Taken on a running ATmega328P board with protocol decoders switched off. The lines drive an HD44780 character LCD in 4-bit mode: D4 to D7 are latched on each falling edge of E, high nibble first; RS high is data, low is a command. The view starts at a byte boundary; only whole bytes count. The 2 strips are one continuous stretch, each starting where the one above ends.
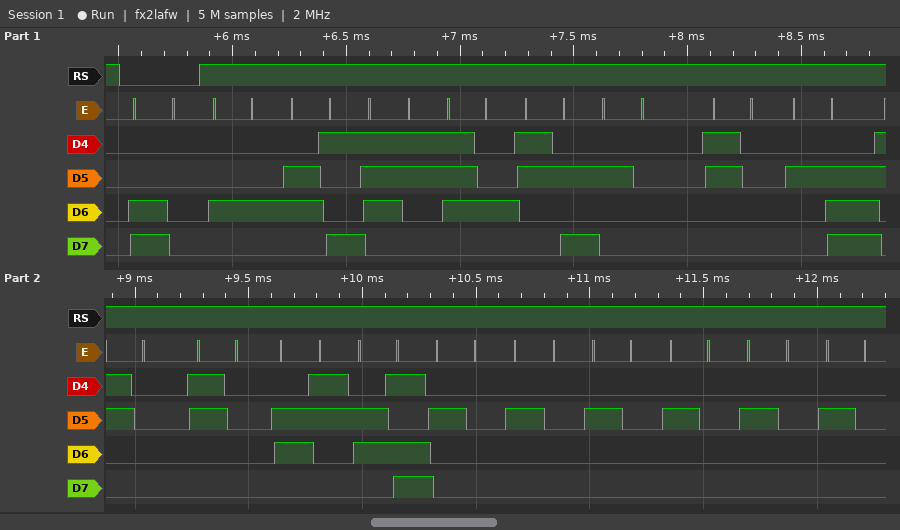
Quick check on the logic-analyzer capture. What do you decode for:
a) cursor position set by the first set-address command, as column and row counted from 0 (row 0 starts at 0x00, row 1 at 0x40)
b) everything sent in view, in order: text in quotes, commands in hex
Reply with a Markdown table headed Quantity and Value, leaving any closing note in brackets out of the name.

| Quantity | Value |
|---|---|
| cursor position set by the first set-address command, as column and row counted from 0 | column 0, row 1 |
| everything sent in view, in order: text in quotes, commands in hex | 0xC0 "Dist: 0.00cm      " |
